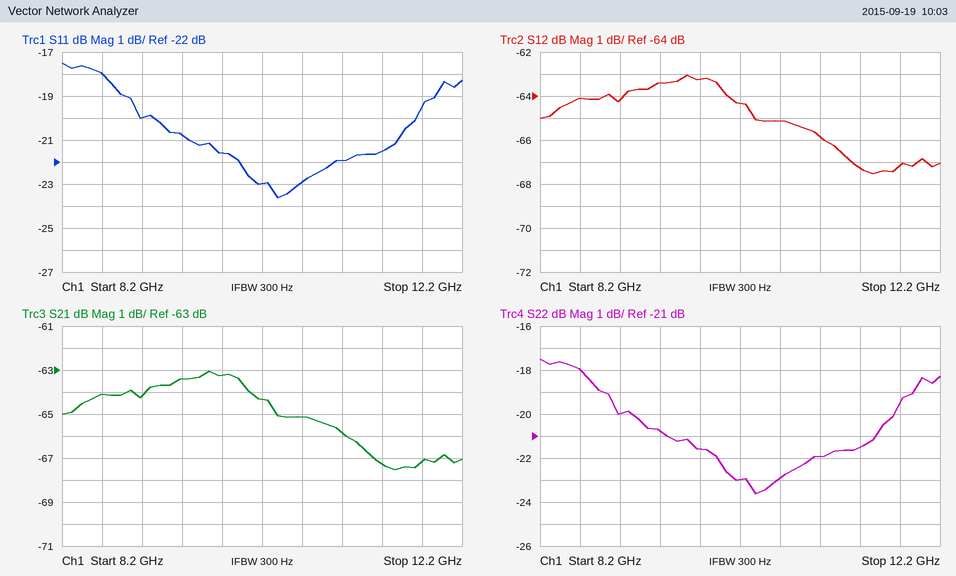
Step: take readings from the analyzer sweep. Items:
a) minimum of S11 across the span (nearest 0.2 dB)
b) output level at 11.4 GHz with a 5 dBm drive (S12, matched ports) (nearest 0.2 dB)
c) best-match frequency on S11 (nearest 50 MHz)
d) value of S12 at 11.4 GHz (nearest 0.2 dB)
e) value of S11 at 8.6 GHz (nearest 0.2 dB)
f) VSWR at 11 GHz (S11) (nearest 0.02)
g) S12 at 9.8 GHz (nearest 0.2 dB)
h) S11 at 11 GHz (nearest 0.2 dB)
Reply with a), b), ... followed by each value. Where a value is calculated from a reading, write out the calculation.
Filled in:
a) -23.6 dB
b) 5 dBm + (-67.2 dB) = -62.2 dBm
c) 10.35 GHz
d) -67.2 dB
e) -18.0 dB
f) |Γ| = 10^(-22/20) = 0.0794; VSWR = (1 + 0.0794)/(1 − 0.0794) ≈ 1.17, so 1.18 to the nearest 0.02
g) -63.2 dB
h) -22.0 dB
